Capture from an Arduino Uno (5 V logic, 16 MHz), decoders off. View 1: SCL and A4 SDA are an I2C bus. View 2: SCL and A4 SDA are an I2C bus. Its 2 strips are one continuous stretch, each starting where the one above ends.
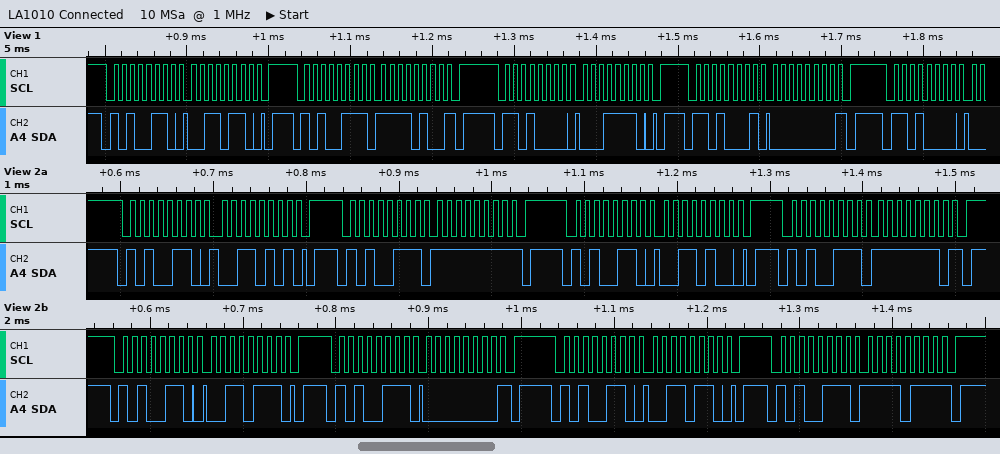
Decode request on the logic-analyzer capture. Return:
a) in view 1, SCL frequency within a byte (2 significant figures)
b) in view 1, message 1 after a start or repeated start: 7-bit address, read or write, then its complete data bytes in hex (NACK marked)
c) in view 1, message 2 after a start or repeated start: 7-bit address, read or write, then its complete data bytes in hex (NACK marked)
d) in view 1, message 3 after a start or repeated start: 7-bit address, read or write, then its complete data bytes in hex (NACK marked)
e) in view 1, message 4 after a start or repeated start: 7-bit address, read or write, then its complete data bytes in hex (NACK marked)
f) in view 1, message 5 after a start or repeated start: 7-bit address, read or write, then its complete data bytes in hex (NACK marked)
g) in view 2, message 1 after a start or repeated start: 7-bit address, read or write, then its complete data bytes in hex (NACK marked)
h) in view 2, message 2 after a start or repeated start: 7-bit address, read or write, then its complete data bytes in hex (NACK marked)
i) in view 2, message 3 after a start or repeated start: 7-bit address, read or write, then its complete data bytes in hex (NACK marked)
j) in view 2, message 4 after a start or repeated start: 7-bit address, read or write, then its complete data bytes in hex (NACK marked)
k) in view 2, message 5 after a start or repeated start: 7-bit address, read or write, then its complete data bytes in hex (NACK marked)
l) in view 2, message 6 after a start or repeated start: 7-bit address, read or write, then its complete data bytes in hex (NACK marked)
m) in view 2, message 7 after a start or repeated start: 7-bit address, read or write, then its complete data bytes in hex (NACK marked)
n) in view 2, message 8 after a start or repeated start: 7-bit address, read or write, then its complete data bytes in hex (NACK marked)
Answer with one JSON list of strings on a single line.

["100 kHz", "0x53 write: 36", "0x53 read: F4 NACK", "0x68 write: 1E", "0x68 read: 00 NACK", "0x68 write", "0x53 write: 35", "0x53 read: FF NACK", "0x53 write: 34", "0x53 read: FE NACK", "0x53 write: 37", "0x53 read: 00 NACK", "0x53 write: 36", "0x53 read: F7 NACK"]
